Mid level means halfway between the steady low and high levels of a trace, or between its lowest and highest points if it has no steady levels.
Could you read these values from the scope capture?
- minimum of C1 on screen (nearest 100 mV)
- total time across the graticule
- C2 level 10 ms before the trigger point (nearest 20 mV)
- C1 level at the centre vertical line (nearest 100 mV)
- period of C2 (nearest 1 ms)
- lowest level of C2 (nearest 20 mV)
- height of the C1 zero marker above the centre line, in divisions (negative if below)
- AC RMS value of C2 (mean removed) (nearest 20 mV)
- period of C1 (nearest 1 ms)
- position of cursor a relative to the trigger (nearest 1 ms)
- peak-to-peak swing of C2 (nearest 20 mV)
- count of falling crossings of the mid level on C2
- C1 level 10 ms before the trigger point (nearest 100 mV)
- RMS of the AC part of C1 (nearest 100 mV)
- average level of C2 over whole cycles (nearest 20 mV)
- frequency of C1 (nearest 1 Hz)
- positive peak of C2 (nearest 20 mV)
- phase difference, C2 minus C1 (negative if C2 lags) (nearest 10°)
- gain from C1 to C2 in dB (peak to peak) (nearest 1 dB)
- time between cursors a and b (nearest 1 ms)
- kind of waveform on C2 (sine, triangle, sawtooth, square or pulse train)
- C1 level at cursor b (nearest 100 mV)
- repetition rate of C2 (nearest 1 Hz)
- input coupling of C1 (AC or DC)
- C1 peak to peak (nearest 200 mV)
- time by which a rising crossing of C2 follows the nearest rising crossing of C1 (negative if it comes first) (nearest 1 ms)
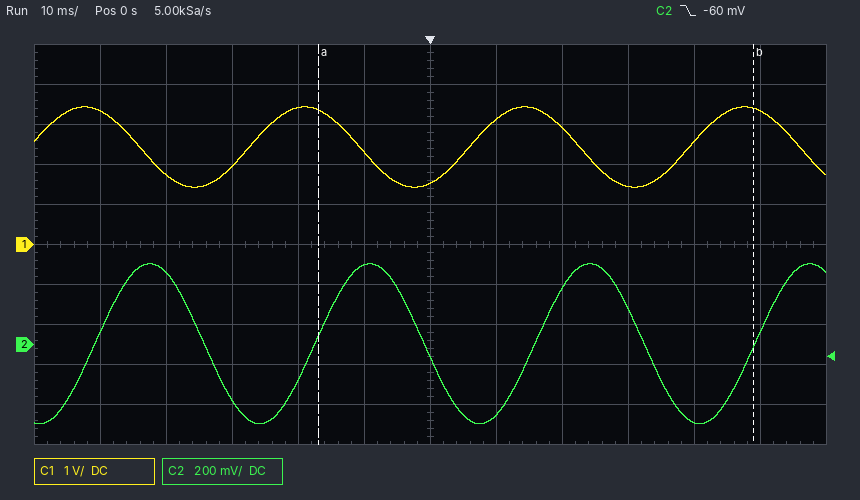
1.4 V
120 ms
400 mV
1.5 V
33 ms
-400 mV
0.0 div
280 mV
33 ms
-17 ms
800 mV
3
2.3 V
700 mV
0 mV
30 Hz
400 mV
-110°
-8 dB
66 ms
sine
3.4 V
30 Hz
DC
2.0 V
+10 ms
